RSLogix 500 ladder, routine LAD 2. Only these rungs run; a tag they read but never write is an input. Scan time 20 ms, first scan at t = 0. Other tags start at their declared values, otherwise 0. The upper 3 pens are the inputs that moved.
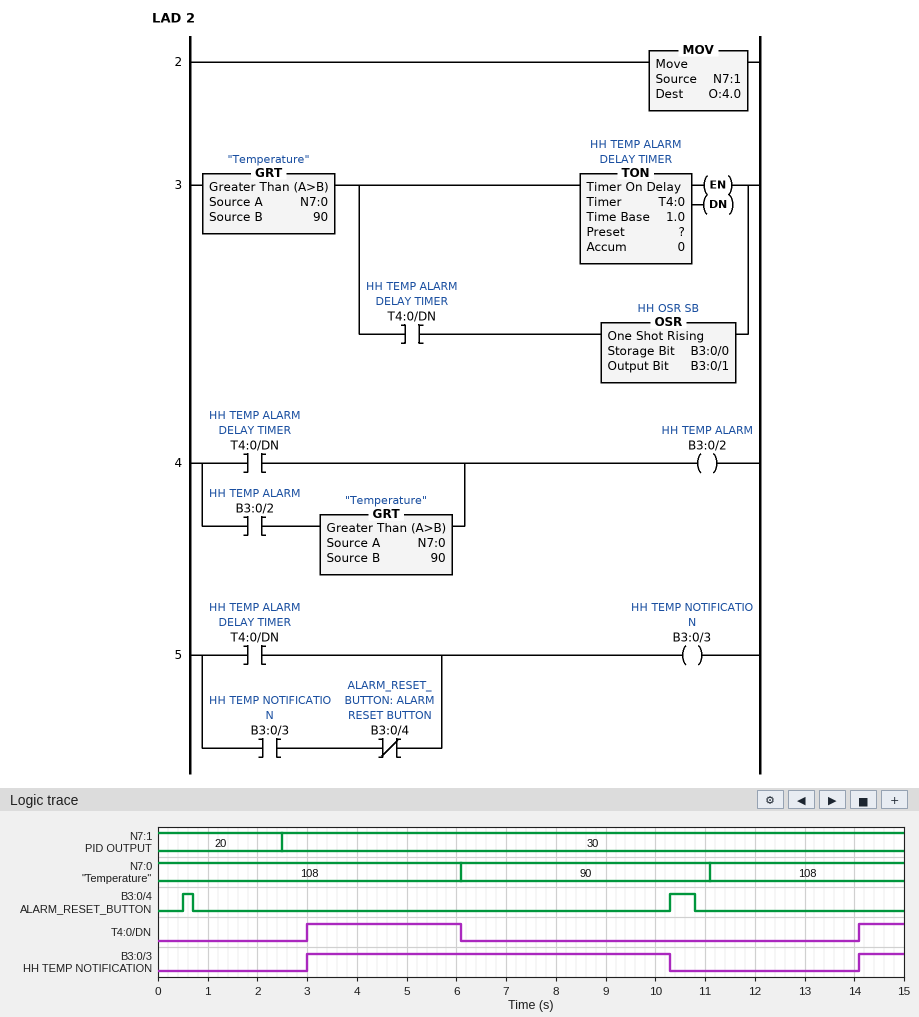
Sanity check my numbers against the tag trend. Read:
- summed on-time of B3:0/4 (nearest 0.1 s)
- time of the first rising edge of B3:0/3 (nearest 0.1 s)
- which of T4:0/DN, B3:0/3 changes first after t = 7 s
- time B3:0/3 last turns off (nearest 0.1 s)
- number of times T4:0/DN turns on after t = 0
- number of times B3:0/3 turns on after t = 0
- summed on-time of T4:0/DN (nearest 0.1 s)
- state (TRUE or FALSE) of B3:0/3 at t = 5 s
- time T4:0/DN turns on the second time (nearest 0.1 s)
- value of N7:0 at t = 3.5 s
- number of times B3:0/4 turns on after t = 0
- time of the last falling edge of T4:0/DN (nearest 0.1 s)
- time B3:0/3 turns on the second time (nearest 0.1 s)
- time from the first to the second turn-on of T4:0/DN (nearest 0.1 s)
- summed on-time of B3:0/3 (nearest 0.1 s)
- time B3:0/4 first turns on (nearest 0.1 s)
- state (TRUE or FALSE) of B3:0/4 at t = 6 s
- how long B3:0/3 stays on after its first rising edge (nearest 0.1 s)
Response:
0.7 s
3.0 s
B3:0/3
10.3 s
2
2
4.0 s
TRUE
14.1 s
108
2
6.1 s
14.1 s
11.1 s
8.2 s
0.5 s
FALSE
7.3 s
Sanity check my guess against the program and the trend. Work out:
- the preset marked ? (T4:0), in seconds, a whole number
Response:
3 s
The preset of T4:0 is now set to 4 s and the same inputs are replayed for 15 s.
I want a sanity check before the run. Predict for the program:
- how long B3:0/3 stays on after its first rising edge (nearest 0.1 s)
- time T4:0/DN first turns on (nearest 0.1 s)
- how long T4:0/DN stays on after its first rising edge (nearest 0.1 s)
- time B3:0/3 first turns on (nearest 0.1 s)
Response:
6.3 s
4.0 s
2.1 s
4.0 s
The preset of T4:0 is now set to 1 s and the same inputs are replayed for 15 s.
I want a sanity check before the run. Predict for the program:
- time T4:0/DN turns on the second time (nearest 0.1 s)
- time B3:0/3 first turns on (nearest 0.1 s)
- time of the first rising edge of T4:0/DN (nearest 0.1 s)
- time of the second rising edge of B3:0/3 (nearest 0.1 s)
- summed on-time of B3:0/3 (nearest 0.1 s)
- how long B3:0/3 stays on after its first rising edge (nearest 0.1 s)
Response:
12.1 s
1.0 s
1.0 s
12.1 s
12.2 s
9.3 s
